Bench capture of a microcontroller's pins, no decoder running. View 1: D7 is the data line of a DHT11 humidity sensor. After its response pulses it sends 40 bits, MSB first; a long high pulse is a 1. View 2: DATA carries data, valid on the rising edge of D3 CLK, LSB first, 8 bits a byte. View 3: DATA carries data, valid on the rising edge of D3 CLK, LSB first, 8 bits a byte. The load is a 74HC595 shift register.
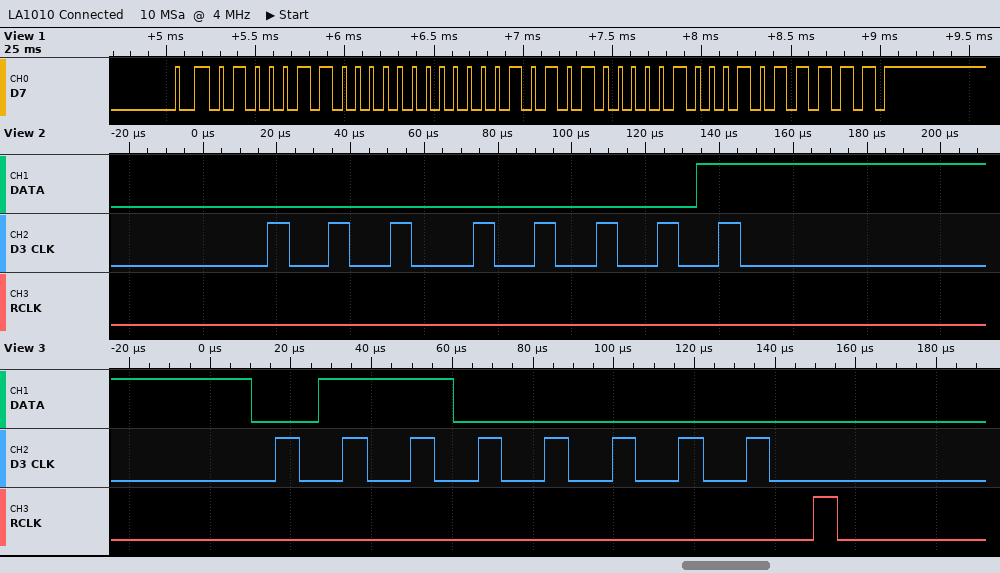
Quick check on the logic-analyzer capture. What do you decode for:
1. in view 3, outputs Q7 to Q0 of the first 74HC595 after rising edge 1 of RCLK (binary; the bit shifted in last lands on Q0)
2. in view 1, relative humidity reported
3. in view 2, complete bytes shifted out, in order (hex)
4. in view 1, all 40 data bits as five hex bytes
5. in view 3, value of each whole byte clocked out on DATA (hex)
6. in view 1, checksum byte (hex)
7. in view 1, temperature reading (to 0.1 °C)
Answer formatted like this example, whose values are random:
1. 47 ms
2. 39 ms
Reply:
1. 01100000
2. 70 %
3. 80
4. 46 00 15 04 5F
5. 0x06
6. 0x5F
7. 21.4 °C
